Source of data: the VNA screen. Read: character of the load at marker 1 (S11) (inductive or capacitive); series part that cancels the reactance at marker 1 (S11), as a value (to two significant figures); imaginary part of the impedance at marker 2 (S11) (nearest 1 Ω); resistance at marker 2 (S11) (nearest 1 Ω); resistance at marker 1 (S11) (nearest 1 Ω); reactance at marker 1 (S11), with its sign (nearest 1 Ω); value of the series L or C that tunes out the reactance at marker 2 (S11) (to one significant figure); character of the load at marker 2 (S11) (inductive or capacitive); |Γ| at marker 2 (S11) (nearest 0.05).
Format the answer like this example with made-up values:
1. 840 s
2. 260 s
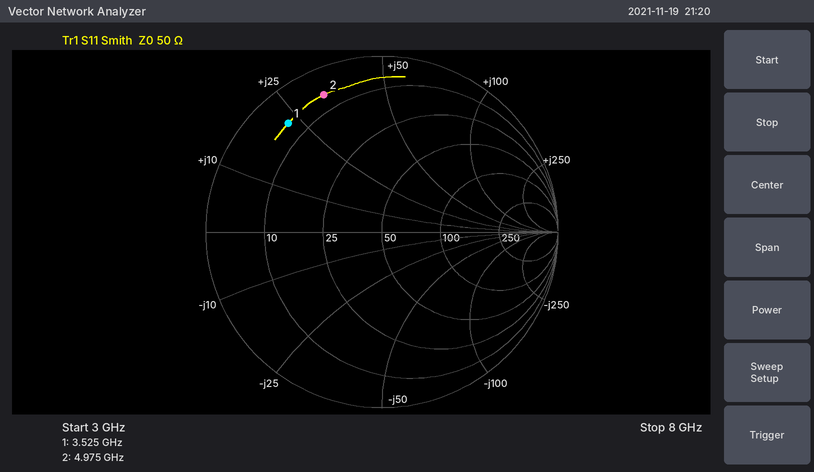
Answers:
1. inductive
2. 2.0 pF
3. +33 Ω
4. 6 Ω
5. 6 Ω
6. +23 Ω
7. 1.0 pF
8. inductive
9. 0.85
